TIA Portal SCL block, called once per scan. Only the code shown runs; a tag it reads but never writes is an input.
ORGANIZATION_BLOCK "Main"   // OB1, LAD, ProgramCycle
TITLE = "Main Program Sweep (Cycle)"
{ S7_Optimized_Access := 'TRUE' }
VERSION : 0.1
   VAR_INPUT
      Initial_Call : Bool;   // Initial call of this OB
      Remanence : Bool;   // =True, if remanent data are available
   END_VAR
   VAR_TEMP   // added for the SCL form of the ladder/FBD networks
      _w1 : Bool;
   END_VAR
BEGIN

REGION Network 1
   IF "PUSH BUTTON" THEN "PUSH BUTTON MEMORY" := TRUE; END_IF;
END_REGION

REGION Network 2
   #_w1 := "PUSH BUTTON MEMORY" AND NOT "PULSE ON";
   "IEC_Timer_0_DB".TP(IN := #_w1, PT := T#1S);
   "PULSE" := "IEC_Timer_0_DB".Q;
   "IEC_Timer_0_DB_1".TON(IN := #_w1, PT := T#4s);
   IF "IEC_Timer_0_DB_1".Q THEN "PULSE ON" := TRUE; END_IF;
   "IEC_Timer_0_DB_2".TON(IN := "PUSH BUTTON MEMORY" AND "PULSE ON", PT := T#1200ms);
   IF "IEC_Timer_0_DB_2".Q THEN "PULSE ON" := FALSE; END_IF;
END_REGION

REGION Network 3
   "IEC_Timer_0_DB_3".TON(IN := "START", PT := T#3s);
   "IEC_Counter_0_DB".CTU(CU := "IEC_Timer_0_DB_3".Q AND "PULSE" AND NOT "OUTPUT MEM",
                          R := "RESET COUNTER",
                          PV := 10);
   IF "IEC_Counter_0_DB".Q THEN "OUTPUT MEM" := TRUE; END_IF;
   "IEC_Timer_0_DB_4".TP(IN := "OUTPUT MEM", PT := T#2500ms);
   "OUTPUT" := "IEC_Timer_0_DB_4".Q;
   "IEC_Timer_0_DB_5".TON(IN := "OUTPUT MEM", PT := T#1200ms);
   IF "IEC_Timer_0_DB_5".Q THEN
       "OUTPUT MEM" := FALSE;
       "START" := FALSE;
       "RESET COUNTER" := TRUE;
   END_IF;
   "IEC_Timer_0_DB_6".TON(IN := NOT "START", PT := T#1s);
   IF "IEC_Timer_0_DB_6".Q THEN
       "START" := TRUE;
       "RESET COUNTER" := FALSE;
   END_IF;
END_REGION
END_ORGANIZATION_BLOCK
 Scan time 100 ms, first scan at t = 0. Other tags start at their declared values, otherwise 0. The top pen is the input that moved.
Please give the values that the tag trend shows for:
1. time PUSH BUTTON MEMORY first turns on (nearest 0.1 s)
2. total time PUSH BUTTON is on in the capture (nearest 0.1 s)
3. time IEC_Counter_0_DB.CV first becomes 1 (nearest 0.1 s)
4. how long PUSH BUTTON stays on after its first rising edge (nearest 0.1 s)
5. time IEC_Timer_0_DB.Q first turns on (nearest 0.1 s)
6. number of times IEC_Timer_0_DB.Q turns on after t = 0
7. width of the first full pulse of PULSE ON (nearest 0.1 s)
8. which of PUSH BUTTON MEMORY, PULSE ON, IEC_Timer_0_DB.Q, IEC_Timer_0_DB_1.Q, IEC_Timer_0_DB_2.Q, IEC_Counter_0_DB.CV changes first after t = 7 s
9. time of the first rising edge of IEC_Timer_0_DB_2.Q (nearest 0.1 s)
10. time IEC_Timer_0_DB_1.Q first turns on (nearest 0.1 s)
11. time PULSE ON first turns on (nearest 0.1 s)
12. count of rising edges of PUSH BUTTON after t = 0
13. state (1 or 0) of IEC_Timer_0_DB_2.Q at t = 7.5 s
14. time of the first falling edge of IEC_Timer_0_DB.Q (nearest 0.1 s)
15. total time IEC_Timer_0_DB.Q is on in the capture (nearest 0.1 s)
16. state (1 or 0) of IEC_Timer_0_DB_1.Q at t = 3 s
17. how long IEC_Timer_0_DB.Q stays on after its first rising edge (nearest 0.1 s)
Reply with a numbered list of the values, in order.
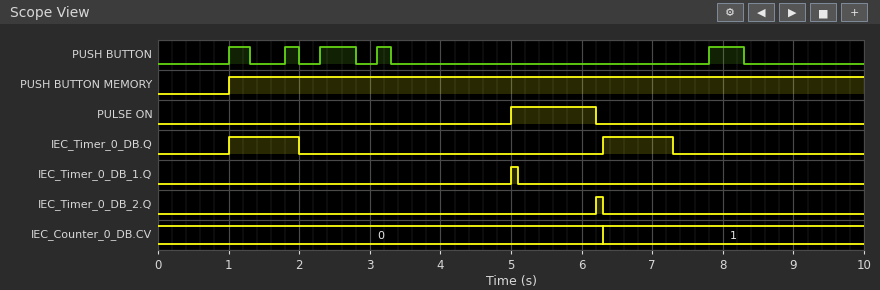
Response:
1. 1.0 s
2. 1.7 s
3. 6.3 s
4. 0.3 s
5. 1.0 s
6. 2
7. 1.2 s
8. IEC_Timer_0_DB.Q
9. 6.2 s
10. 5.0 s
11. 5.0 s
12. 5
13. 0
14. 2.0 s
15. 2.0 s
16. 0
17. 1.0 s
